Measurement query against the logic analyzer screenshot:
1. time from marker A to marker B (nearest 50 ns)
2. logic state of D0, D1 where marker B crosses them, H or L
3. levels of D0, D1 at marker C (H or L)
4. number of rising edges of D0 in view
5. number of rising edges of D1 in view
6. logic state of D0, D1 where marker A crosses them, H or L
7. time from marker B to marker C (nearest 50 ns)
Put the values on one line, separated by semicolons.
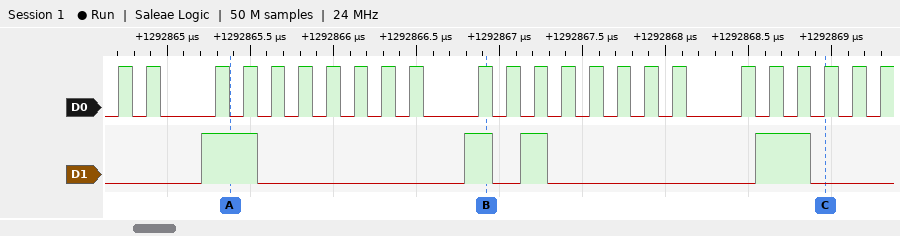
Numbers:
1550 ns; D0=H, D1=H; D0=H, D1=L; 24; 4; D0=L, D1=H; 2050 ns
